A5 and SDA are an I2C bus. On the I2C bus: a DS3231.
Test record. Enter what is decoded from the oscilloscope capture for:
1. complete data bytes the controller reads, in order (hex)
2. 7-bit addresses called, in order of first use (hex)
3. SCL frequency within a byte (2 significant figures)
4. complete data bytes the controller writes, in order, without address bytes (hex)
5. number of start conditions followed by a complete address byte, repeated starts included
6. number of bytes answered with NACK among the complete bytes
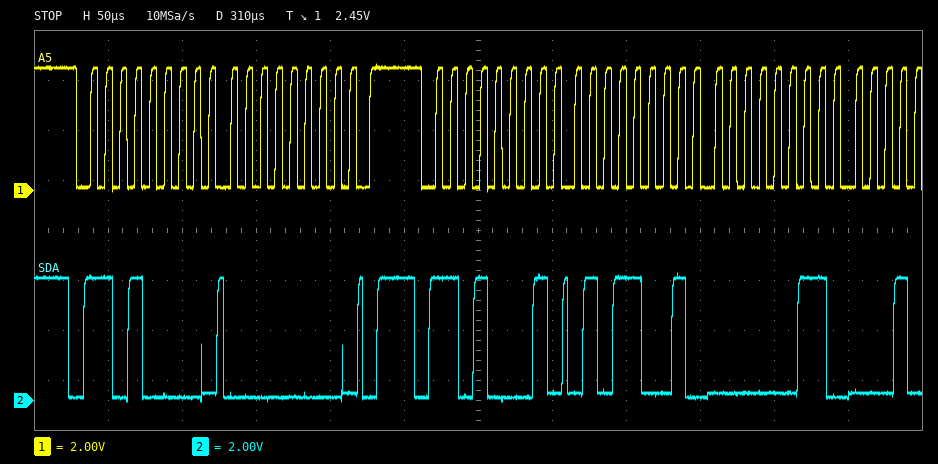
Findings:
59 03
0x68
100 kHz
00
2
0
